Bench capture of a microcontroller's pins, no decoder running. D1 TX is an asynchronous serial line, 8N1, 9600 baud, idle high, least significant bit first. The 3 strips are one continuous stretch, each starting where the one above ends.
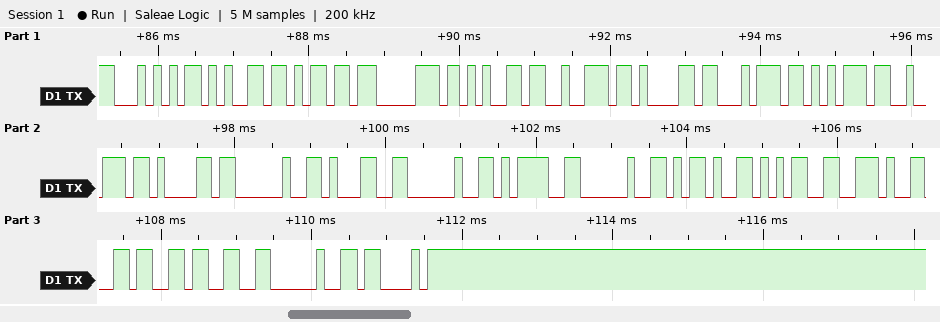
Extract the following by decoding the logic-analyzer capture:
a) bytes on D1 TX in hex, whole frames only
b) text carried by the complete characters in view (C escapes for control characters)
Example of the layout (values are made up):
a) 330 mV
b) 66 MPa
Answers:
a) 54 65 6D 70 65 72 61 74 75 72 61 20 31 20 3D 20 2D 35 2E 36 33 20 43
b) "Temperatura 1 = -5.63 C"
